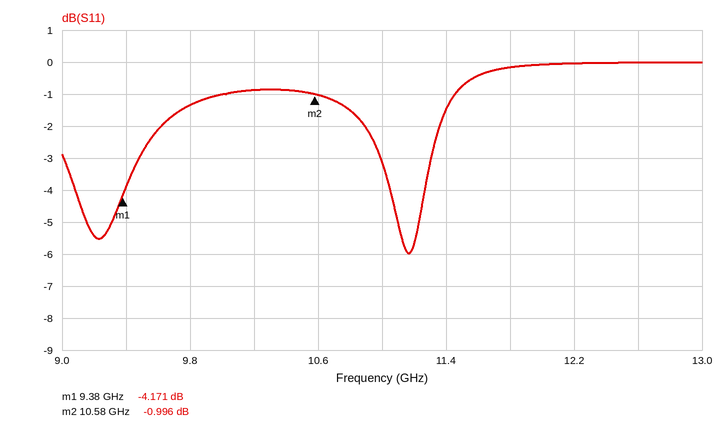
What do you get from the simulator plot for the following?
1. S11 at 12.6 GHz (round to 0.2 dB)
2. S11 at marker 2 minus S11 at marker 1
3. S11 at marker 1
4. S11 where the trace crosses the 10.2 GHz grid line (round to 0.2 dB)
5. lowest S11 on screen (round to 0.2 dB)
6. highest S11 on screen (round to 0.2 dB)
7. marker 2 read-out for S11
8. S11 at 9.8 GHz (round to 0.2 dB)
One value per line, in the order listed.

0.0 dB
3.175 dB
-4.171 dB
-0.8 dB
-6.0 dB
0.0 dB
-0.996 dB
-1.4 dB
